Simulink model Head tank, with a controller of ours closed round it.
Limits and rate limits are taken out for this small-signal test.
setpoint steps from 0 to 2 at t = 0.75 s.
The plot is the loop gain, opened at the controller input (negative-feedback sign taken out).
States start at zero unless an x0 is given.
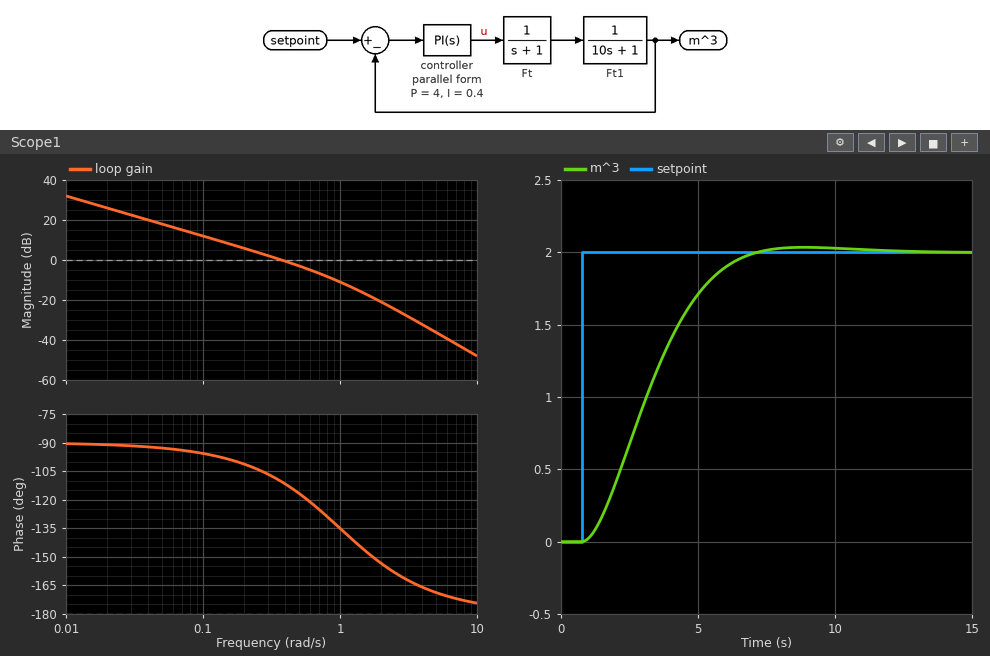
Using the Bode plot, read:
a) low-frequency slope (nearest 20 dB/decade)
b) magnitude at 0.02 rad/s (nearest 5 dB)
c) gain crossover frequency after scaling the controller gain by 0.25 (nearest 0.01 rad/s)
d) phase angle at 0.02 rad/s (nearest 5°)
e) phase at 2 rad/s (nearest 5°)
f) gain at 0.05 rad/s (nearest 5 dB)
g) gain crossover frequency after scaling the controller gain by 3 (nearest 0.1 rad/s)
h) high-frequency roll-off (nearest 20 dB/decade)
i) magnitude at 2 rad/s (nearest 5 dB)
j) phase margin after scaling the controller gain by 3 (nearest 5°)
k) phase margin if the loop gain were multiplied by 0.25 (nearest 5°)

-20 dB/decade
25 dB
0.10 rad/s
-90°
-155°
20 dB
0.9 rad/s
-40 dB/decade
-20 dB
50°
85°
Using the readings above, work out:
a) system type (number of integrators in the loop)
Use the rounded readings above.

1
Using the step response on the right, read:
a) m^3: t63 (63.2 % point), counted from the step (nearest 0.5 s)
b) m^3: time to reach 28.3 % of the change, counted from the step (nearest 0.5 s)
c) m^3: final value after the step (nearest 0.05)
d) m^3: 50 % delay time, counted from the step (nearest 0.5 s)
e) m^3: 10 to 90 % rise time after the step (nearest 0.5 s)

3.0 s
1.5 s
2.00
2.5 s
4.0 s
